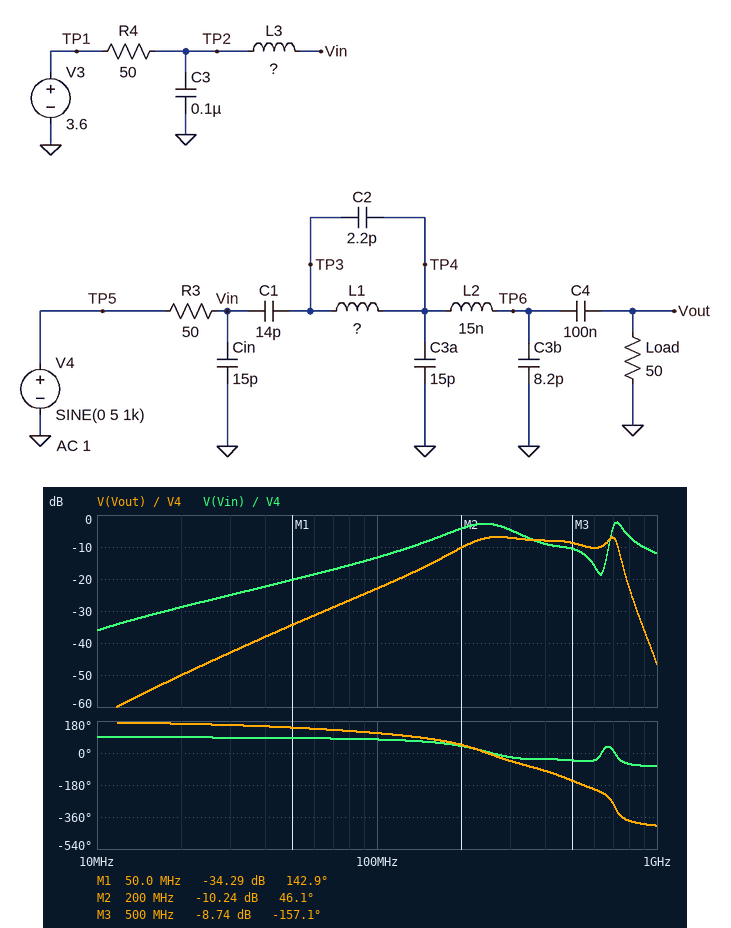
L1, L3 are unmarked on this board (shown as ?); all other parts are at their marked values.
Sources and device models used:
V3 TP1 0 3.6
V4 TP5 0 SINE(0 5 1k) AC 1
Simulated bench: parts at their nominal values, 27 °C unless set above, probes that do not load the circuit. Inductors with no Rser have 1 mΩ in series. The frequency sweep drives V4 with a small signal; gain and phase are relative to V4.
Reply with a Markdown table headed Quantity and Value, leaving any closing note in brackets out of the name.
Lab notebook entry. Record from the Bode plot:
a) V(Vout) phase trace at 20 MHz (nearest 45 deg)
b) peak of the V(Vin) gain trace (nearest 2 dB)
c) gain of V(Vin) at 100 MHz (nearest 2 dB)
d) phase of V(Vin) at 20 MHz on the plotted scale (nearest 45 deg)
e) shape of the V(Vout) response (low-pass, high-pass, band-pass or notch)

| Quantity | Value |
|---|---|
| V(Vout) phase trace at 20 MHz | 180 deg |
| peak of the V(Vin) gain trace | -2 dB |
| gain of V(Vin) at 100 MHz | -14 dB |
| phase of V(Vin) at 20 MHz on the plotted scale | 90 deg |
| shape of the V(Vout) response | band-pass |
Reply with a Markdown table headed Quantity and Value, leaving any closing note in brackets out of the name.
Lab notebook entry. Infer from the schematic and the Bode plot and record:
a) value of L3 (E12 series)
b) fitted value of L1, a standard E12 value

| Quantity | Value |
|---|---|
| value of L3 | 15 nH |
| fitted value of L1, a standard E12 value | 8.2 nH |
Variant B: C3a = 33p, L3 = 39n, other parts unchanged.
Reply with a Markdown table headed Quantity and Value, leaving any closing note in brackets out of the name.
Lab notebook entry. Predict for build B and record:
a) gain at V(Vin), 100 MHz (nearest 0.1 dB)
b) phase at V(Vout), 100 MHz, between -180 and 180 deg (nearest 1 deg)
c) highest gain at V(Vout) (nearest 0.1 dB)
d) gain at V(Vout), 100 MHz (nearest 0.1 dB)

| Quantity | Value |
|---|---|
| gain at V(Vin), 100 MHz | -4.1 dB |
| phase at V(Vout), 100 MHz, between -180 and 180 deg | 72 deg |
| highest gain at V(Vout) | -9.9 dB |
| gain at V(Vout), 100 MHz | -16.1 dB |
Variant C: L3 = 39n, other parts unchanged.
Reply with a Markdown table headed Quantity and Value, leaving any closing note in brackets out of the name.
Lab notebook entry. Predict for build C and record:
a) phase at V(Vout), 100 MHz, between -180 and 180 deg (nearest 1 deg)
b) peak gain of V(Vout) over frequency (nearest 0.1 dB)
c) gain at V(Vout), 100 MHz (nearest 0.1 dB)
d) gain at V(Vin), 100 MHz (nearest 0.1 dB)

| Quantity | Value |
|---|---|
| phase at V(Vout), 100 MHz, between -180 and 180 deg | 83 deg |
| peak gain of V(Vout) over frequency | -6.3 dB |
| gain at V(Vout), 100 MHz | -14.0 dB |
| gain at V(Vin), 100 MHz | -4.3 dB |
